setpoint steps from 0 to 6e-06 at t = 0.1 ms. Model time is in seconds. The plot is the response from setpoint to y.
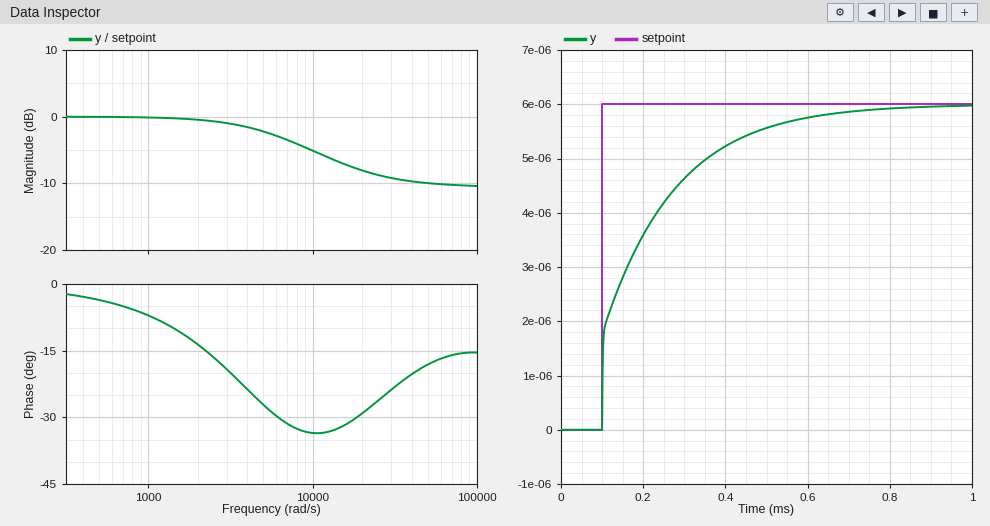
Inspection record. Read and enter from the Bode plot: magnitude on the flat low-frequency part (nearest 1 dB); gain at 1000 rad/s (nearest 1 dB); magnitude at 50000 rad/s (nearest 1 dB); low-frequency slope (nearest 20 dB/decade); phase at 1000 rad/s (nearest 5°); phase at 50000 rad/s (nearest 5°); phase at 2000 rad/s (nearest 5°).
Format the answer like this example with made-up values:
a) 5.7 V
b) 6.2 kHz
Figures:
a) 0 dB
b) 0 dB
c) -10 dB
d) 0 dB/decade
e) -5°
f) -20°
g) -15°
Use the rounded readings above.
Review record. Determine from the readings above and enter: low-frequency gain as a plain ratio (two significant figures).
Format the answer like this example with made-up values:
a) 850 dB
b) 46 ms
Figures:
a) 1.0
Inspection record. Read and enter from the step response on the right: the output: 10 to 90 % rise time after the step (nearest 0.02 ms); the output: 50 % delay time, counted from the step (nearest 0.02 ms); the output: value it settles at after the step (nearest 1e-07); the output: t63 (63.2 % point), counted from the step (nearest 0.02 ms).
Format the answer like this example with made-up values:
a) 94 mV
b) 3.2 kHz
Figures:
a) 0.34 ms
b) 0.06 ms
c) 0.0000060
d) 0.12 ms
